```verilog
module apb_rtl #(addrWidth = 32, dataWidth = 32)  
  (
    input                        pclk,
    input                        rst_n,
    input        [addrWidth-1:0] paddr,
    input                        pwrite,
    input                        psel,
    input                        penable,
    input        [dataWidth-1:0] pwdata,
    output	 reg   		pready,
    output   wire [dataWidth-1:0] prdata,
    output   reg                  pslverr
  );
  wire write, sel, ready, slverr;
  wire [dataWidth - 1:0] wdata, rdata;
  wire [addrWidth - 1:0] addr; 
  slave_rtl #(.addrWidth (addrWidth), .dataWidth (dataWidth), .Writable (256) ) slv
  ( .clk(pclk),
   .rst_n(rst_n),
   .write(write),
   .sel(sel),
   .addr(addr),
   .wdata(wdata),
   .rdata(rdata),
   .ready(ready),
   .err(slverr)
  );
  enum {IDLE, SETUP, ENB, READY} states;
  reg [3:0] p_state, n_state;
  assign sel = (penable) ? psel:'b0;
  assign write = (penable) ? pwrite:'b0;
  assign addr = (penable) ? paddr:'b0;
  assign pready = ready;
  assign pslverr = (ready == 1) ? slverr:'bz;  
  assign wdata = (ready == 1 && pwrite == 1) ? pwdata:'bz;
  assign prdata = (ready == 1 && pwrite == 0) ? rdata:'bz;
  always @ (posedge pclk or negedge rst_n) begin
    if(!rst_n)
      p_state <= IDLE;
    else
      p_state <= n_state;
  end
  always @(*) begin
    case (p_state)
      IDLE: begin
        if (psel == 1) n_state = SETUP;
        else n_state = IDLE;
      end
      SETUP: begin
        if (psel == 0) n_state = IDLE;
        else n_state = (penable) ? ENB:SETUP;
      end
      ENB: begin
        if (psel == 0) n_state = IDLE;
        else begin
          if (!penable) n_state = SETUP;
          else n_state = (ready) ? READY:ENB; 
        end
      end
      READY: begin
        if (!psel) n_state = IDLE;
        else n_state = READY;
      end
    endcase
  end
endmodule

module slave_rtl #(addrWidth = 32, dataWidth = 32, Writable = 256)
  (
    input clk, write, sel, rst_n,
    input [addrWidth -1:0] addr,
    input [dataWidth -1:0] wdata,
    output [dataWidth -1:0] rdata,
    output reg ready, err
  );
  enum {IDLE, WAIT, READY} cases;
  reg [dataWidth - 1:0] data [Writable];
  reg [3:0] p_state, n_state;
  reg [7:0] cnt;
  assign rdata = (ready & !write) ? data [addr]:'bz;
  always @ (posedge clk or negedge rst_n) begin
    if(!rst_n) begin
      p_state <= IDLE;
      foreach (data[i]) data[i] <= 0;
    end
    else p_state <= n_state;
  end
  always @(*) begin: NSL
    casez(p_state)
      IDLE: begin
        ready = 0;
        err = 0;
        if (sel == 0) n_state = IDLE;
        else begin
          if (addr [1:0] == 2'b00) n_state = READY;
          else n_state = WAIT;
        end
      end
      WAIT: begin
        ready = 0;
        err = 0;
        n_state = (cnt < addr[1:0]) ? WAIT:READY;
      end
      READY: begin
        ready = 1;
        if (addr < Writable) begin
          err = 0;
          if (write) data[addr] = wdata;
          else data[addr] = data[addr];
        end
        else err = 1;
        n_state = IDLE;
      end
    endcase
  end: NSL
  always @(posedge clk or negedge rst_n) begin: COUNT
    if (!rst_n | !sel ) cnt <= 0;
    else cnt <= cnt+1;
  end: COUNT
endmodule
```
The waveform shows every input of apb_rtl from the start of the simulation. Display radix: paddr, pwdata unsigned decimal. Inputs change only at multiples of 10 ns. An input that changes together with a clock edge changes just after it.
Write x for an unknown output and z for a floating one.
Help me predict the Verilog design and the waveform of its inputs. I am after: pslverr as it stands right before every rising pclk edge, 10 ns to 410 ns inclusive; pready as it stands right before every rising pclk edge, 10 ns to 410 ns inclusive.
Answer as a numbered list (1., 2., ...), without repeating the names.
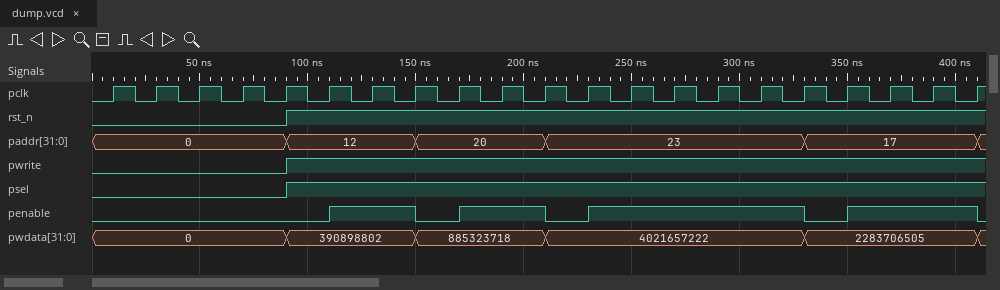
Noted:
1. z z z z z z z 0 z z 0 z z z z z 0 z z z 0
2. 0 0 0 0 0 0 0 1 0 0 1 0 0 0 0 0 1 0 0 0 1
